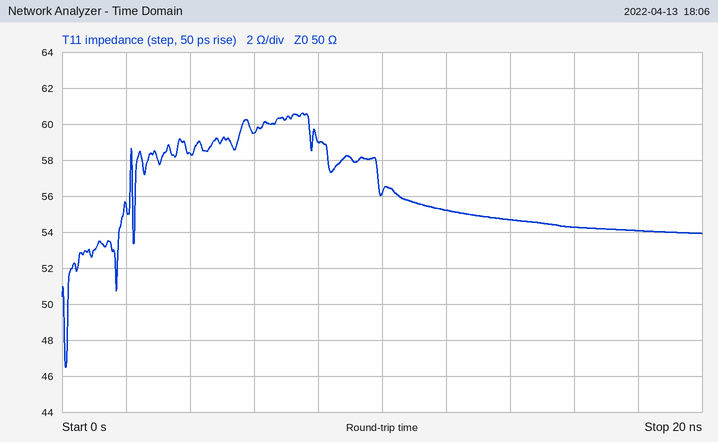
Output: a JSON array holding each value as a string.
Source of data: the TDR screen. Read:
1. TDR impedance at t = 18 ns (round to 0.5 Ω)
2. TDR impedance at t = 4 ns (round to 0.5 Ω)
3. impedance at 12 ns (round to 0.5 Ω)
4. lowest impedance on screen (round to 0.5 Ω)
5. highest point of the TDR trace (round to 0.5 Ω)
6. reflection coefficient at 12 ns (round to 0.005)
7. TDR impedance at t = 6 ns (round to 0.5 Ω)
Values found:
["54.0 Ω", "58.5 Ω", "55.0 Ω", "46.5 Ω", "60.5 Ω", "+0.050", "59.5 Ω"]
